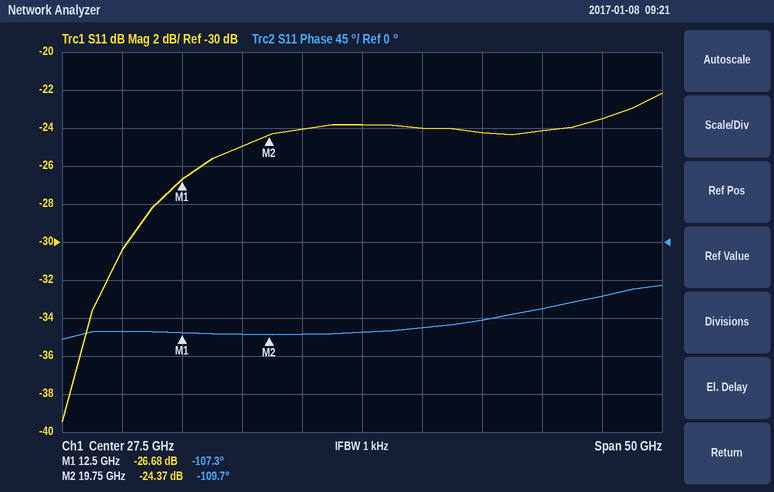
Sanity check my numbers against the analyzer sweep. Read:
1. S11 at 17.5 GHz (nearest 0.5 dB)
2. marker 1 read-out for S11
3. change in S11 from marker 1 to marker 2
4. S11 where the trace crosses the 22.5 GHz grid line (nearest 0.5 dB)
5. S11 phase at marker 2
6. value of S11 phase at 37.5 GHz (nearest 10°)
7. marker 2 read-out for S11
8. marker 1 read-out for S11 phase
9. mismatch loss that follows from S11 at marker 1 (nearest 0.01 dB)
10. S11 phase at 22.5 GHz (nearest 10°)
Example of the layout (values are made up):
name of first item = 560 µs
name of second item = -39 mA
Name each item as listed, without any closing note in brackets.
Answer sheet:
S11 at 17.5 GHz = -25.0 dB
marker 1 read-out for S11 = -26.68 dB
change in S11 from marker 1 to marker 2 = 2.31 dB
S11 where the trace crosses the 22.5 GHz grid line = -24.0 dB
S11 phase at marker 2 = -109.7°
value of S11 phase at 37.5 GHz = -90°
marker 2 read-out for S11 = -24.37 dB
marker 1 read-out for S11 phase = -107.3°
mismatch loss that follows from S11 at marker 1 = 0.01 dB
S11 phase at 22.5 GHz = -110°
